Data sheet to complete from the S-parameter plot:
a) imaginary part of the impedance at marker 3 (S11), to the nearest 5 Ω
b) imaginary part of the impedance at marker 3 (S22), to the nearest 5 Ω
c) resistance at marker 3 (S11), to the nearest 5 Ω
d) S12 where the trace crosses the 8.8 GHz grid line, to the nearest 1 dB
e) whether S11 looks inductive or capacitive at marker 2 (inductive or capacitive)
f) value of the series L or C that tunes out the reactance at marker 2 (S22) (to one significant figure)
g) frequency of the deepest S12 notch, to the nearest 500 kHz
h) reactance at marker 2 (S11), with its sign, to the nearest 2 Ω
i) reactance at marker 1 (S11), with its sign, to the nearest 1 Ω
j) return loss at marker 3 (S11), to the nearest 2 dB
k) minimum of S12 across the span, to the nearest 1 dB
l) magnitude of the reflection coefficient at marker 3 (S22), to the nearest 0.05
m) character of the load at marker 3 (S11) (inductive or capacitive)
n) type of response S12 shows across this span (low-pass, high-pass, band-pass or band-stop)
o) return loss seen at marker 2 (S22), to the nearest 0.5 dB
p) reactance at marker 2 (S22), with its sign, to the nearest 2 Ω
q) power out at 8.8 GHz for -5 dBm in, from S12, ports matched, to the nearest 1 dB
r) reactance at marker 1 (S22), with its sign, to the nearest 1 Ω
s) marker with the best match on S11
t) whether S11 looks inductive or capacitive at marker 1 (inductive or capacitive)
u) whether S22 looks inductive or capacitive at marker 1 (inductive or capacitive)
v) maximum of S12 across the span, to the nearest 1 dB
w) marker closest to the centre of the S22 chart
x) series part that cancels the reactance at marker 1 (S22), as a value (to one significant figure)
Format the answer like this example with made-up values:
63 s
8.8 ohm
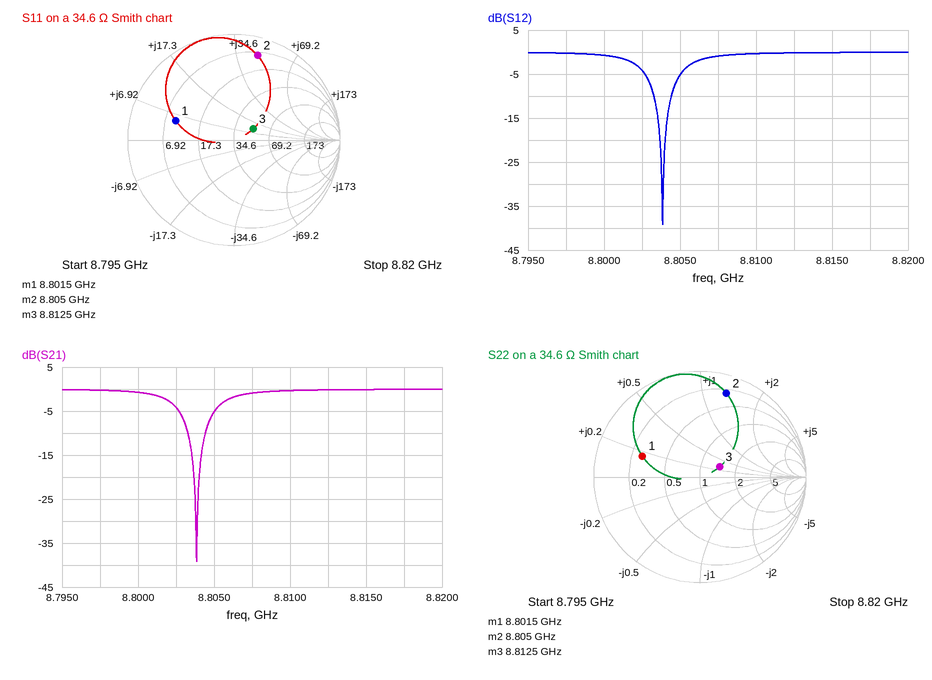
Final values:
+10 Ω
+10 Ω
50 Ω
-1 dB
inductive
400 fF
8.8040 GHz
+44 Ω
+5 Ω
14 dB
-39 dB
0.20
inductive
band-stop
1.5 dB
+46 Ω
-6 dBm
+6 Ω
marker 3
inductive
inductive
0 dB
marker 3
3 pF
